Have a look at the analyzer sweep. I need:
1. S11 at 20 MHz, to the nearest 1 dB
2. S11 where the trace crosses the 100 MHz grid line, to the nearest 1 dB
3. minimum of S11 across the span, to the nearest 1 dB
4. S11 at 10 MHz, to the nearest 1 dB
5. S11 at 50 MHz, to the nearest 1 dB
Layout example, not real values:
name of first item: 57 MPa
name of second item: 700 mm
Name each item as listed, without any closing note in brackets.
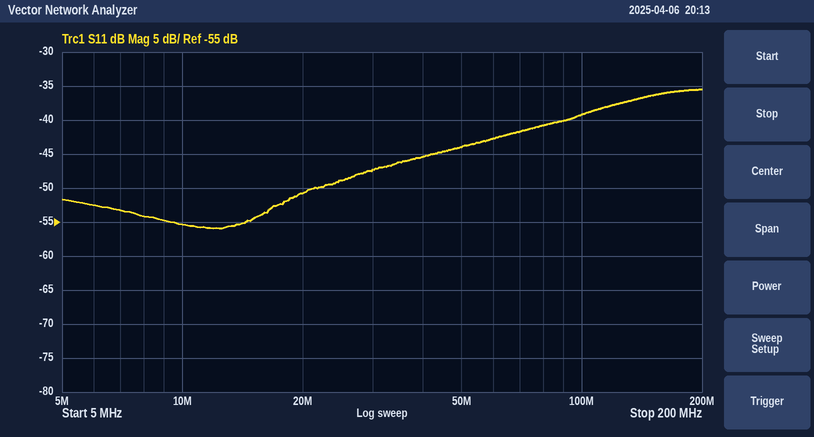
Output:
S11 at 20 MHz, to the nearest 1 dB: -51 dB
S11 where the trace crosses the 100 MHz grid line, to the nearest 1 dB: -39 dB
minimum of S11 across the span, to the nearest 1 dB: -56 dB
S11 at 10 MHz, to the nearest 1 dB: -55 dB
S11 at 50 MHz, to the nearest 1 dB: -44 dB
